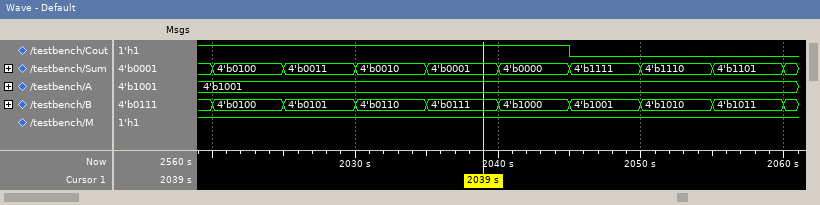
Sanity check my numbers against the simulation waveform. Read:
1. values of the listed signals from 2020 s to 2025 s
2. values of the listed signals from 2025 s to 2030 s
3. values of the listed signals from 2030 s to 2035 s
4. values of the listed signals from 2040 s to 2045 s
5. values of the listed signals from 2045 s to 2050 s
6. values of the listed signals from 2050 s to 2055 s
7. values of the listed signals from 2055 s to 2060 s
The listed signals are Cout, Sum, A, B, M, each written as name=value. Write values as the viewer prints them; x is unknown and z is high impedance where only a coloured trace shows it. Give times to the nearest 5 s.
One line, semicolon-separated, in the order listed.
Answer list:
Cout=1, Sum=4'b0100, A=4'b1001, B=4'b0100, M=1; Cout=1, Sum=4'b0011, A=4'b1001, B=4'b0101, M=1; Cout=1, Sum=4'b0010, A=4'b1001, B=4'b0110, M=1; Cout=1, Sum=4'b0000, A=4'b1001, B=4'b1000, M=1; Cout=0, Sum=4'b1111, A=4'b1001, B=4'b1001, M=1; Cout=0, Sum=4'b1110, A=4'b1001, B=4'b1010, M=1; Cout=0, Sum=4'b1101, A=4'b1001, B=4'b1011, M=1
